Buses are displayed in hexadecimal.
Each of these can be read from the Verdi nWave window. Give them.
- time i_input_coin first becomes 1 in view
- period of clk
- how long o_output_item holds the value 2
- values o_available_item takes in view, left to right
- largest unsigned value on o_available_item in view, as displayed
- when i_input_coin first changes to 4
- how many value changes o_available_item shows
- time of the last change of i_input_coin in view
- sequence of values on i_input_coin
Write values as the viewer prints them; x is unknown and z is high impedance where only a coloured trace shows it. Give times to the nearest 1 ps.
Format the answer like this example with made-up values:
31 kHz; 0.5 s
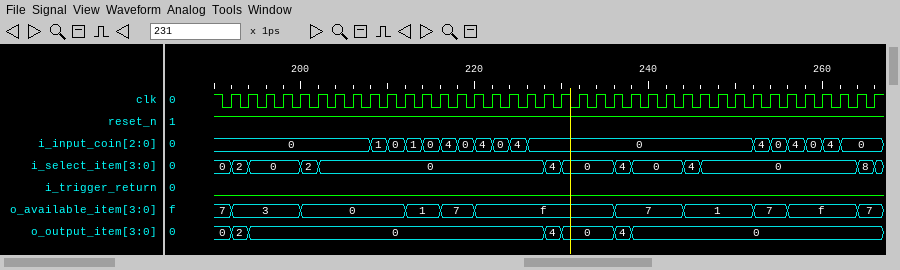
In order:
208 ps; 2 ps; 2 ps; 7, 3, 0, 1, 7, f, 7, 1, 7, f, 7; f; 216 ps; 10; 262 ps; 0, 1, 0, 1, 0, 4, 0, 4, 0, 4, 0, 4, 0, 4, 0, 4, 0
